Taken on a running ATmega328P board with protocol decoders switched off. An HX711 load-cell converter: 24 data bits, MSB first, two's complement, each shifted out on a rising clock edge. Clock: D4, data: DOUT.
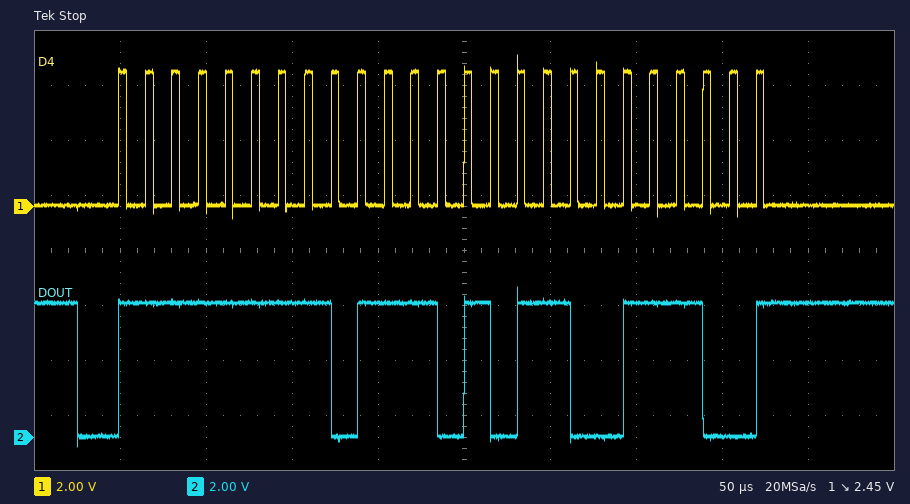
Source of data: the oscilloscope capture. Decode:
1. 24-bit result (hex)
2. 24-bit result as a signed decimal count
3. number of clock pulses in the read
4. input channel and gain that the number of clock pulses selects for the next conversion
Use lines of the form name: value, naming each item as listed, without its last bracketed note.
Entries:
24-bit result: 0xFF759C
24-bit result as a signed decimal count: -35428
number of clock pulses in the read: 25
input channel and gain that the number of clock pulses selects for the next conversion: channel A, gain 128
